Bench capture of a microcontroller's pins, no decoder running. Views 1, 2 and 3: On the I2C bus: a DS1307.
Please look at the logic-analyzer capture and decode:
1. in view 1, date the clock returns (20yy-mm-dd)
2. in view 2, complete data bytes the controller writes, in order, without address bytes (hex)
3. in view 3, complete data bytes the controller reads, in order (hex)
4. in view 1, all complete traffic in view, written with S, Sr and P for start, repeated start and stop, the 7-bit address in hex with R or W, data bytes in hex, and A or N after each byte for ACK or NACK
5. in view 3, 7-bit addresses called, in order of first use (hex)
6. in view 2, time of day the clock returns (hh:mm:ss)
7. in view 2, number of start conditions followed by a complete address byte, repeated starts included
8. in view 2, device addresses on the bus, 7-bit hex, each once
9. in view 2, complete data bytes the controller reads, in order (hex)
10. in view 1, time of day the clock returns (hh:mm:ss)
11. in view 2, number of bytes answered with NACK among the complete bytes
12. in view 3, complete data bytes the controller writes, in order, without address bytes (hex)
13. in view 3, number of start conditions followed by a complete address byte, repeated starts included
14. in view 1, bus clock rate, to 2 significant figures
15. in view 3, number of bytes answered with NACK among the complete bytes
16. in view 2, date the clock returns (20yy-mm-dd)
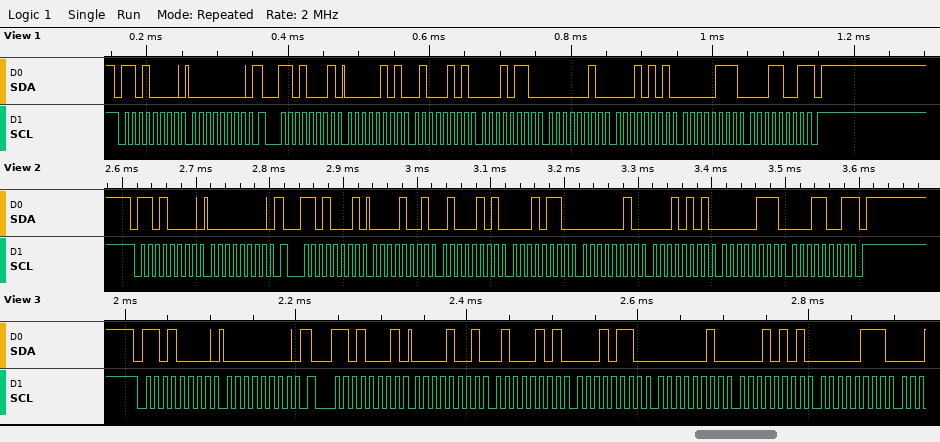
2019-07-15
00
09 45 16 02 15 07
S 68W A 00 A Sr 68R A 05 A 45 A 16 A 02 A 15 A 07 A 19 N P
0x68
16:45:09
2
0x68
09 45 16 02 15 07 19
16:45:05
1
00
2
100 kHz
0
2019-07-15
